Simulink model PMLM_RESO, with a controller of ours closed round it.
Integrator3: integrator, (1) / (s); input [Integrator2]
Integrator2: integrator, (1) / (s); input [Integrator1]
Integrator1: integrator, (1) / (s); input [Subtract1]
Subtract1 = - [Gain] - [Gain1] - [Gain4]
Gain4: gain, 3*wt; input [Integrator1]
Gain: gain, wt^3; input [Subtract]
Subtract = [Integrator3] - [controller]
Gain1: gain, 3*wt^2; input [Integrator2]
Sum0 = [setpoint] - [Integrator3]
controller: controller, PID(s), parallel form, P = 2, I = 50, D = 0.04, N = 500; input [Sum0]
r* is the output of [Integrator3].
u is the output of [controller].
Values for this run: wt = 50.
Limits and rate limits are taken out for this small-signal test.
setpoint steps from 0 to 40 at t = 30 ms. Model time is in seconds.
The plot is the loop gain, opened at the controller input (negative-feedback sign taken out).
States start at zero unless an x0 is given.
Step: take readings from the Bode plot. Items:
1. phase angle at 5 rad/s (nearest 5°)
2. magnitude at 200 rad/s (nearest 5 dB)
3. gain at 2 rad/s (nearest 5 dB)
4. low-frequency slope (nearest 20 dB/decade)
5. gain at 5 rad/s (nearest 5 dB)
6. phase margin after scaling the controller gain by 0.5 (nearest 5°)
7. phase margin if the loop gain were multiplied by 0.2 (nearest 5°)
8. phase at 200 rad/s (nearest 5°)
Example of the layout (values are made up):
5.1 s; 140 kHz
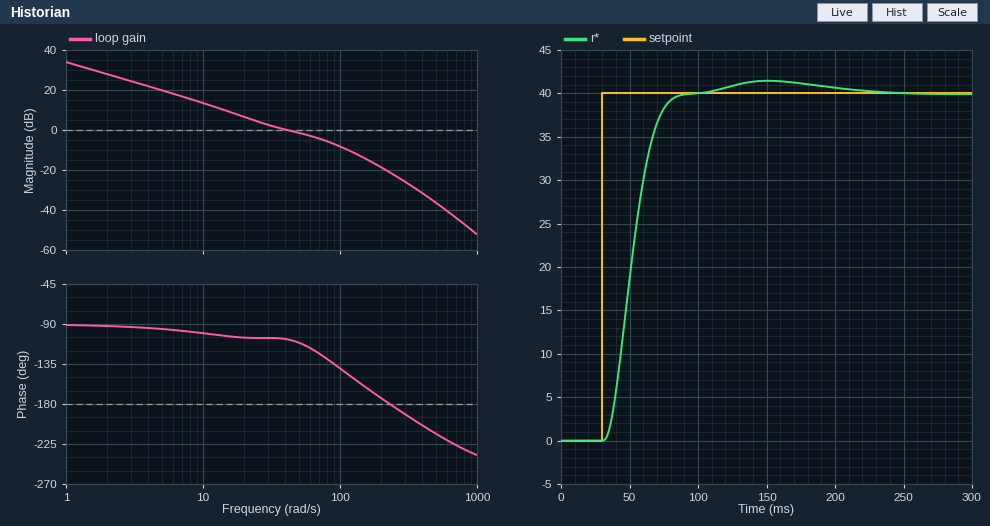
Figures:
-95°; -20 dB; 30 dB; -20 dB/decade; 20 dB; 75°; 80°; -175°
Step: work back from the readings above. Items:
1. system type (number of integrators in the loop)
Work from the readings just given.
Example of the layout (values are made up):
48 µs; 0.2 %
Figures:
1
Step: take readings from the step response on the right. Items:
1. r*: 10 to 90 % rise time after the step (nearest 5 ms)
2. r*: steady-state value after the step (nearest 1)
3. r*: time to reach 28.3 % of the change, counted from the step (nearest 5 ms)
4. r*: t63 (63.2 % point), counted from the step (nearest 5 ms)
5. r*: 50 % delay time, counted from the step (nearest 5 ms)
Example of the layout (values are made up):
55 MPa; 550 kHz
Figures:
30 ms; 40; 15 ms; 25 ms; 20 ms
